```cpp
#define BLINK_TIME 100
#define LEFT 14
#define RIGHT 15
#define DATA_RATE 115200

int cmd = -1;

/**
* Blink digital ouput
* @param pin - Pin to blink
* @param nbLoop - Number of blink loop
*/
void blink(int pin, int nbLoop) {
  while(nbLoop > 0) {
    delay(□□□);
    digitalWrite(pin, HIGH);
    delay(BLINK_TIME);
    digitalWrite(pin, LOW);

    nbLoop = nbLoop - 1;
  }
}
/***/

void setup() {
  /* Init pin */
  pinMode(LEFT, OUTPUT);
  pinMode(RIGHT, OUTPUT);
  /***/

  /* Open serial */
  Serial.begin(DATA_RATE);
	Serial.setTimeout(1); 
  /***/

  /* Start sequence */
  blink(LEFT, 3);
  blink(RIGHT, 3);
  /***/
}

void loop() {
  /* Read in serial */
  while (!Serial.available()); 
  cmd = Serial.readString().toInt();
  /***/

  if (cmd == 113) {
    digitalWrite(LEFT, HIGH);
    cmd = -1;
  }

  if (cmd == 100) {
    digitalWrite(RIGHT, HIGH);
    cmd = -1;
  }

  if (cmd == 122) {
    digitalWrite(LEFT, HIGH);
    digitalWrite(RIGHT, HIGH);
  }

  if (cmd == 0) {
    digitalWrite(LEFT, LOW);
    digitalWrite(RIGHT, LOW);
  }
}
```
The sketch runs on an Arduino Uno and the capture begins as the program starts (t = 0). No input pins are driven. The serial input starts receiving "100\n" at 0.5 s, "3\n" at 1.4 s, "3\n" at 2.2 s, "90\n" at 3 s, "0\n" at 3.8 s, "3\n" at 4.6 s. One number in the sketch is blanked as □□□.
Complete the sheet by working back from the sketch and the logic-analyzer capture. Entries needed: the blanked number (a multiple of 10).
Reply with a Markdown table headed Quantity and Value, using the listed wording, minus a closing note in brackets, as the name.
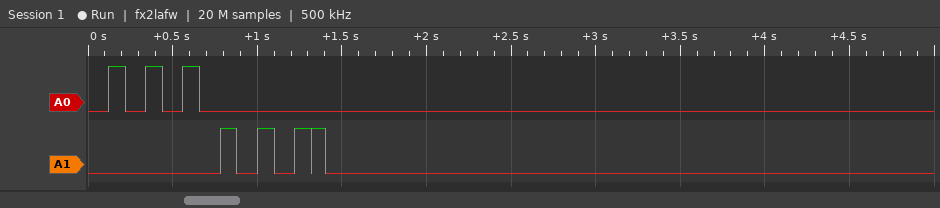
| Quantity | Value |
|---|---|
| the blanked number | 120 |
